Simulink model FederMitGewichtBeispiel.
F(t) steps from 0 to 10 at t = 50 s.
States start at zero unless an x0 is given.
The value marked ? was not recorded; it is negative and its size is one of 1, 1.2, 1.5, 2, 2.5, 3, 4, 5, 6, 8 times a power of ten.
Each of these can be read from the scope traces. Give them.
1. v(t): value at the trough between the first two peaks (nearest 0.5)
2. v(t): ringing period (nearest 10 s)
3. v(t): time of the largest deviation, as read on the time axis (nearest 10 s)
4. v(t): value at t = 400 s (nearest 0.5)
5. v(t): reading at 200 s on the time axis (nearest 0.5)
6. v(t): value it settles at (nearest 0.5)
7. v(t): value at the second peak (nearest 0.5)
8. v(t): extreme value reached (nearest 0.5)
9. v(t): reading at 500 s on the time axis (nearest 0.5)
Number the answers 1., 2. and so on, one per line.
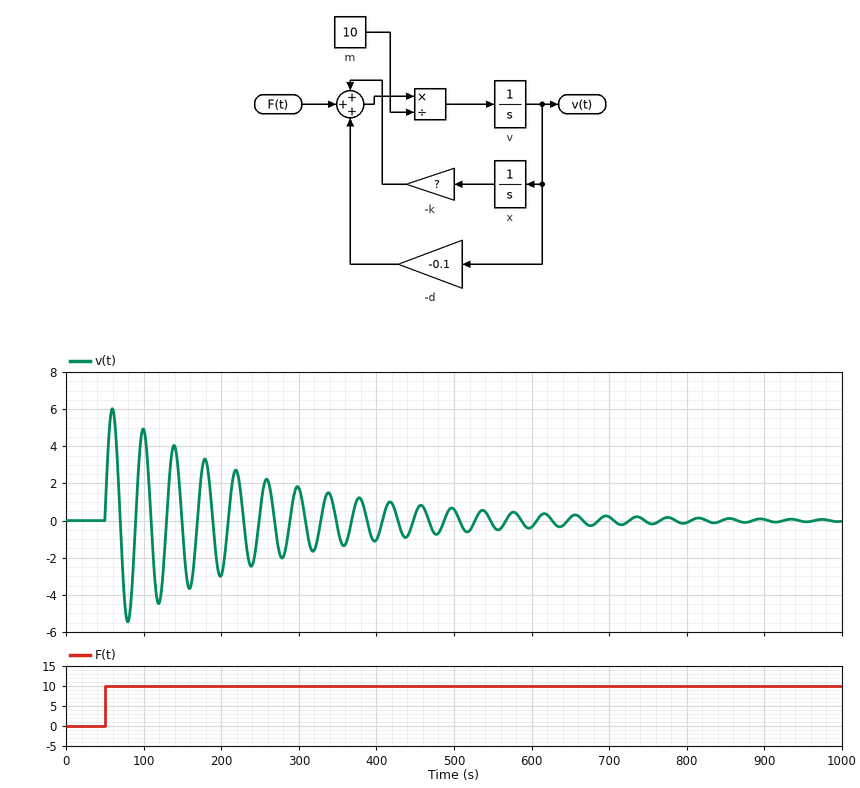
1. -5.5
2. 40 s
3. 60 s
4. -1.0
5. -3.0
6. 0.0
7. 5.0
8. 6.0
9. 0.5
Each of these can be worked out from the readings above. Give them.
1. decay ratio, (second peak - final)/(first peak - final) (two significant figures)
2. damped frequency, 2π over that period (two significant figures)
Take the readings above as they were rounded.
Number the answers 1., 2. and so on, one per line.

1. 0.83
2. 0.16 rad/s
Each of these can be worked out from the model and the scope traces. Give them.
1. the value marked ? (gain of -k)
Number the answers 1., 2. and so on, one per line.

1. -0.25
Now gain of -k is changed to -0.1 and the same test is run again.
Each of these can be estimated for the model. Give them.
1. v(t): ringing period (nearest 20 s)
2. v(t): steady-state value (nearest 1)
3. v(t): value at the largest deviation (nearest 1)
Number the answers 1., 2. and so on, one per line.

1. 60 s
2. 0
3. 9
